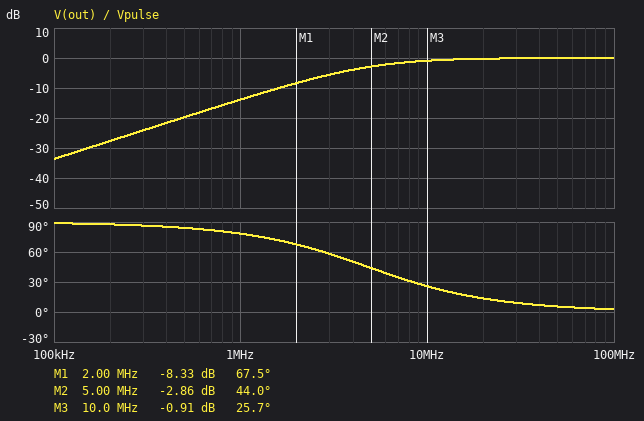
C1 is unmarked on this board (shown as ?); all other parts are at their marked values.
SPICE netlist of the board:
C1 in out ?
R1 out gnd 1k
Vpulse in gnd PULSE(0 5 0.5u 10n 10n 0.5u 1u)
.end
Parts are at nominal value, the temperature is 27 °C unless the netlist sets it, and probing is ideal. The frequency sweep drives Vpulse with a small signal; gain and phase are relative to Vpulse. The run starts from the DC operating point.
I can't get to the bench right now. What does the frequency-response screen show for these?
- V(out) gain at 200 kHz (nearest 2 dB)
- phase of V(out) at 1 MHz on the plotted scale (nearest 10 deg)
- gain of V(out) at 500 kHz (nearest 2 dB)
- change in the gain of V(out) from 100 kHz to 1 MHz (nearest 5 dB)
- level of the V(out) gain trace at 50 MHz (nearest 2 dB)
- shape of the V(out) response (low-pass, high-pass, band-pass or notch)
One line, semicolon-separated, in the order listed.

-28 dB; 80 deg; -20 dB; 20 dB; 0 dB; high-pass
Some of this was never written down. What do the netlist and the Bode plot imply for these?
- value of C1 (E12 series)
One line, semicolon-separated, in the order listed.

33 pF
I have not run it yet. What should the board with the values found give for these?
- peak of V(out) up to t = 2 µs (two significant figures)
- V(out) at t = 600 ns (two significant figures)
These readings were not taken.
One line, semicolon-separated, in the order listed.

4.3 V; 280 mV
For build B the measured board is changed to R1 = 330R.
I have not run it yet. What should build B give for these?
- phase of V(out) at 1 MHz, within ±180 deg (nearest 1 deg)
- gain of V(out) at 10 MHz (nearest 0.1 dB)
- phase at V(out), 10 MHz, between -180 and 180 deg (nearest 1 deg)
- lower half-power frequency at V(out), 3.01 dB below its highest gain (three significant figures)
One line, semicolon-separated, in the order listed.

86 deg; -5.0 dB; 56 deg; 14.6 MHz
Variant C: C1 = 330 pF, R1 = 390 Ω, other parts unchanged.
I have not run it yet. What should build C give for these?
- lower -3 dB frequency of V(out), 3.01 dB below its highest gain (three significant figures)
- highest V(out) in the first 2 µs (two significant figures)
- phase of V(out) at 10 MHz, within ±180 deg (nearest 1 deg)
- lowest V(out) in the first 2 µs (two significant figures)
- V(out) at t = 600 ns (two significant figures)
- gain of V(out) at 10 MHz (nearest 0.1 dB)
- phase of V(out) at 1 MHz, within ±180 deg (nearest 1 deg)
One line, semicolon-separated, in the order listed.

1.24 MHz; 4.8 V; 7 deg; -4.7 V; 2.4 V; -0.1 dB; 51 deg
